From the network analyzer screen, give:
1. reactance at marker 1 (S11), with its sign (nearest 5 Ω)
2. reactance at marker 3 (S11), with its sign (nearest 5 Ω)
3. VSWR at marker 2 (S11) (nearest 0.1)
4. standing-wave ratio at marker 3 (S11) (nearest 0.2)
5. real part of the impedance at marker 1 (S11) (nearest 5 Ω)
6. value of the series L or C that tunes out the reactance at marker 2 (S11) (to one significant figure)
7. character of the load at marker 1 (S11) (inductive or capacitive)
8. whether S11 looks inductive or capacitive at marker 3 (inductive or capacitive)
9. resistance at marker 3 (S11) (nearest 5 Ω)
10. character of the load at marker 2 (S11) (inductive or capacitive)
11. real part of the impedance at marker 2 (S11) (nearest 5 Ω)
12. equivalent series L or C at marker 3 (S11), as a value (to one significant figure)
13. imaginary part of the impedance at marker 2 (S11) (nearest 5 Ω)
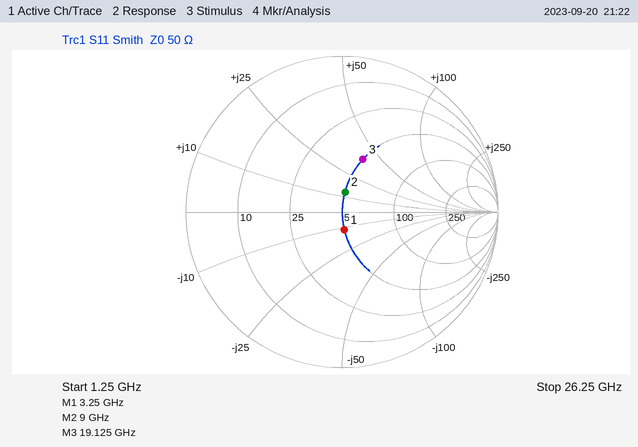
-10 Ω
+40 Ω
1.3
2.2
50 Ω
1 pF
capacitive
inductive
50 Ω
inductive
50 Ω
300 pH
+15 Ω
